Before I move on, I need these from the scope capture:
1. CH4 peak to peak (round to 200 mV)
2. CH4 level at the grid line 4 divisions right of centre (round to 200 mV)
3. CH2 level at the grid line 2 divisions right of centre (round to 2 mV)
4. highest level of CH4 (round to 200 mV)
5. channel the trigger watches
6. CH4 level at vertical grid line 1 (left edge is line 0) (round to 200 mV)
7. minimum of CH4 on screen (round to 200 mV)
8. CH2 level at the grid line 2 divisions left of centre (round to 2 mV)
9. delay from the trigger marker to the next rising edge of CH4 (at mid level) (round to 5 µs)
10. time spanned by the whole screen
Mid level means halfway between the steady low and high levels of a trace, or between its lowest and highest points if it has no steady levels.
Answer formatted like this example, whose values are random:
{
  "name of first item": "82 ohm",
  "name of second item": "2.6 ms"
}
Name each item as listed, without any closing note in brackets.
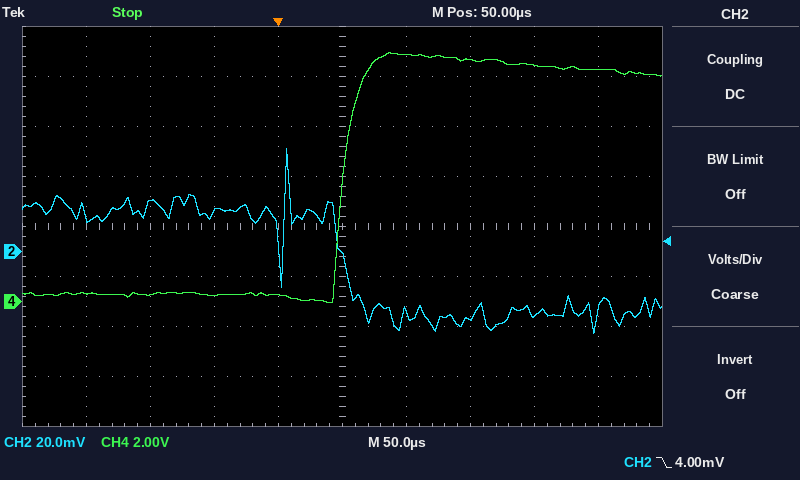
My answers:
{
  "CH4 peak to peak": "10.0 V",
  "CH4 level at the grid line 4 divisions right of centre": "9.2 V",
  "CH2 level at the grid line 2 divisions right of centre": "-26 mV",
  "highest level of CH4": "10.0 V",
  "channel the trigger watches": "CH2",
  "CH4 level at vertical grid line 1 (left edge is line 0)": "400 mV",
  "minimum of CH4 on screen": "0.0 V",
  "CH2 level at the grid line 2 divisions left of centre": "16 mV",
  "delay from the trigger marker to the next rising edge of CH4 (at mid level)": "50 µs",
  "time spanned by the whole screen": "500 µs"
}
